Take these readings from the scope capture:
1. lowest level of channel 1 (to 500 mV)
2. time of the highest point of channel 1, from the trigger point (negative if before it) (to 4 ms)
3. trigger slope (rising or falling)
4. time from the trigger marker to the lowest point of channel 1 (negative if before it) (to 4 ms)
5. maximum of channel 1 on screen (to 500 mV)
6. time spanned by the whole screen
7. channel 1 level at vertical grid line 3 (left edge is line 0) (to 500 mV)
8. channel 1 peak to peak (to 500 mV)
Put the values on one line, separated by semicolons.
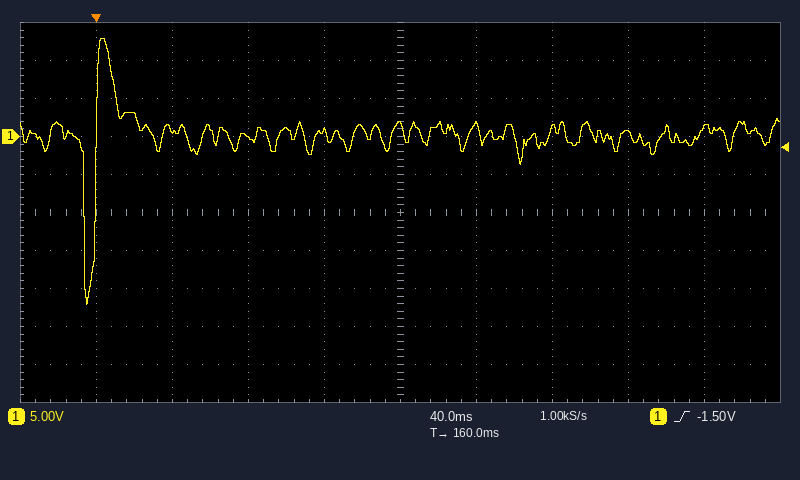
-22.0 V; +4 ms; rising; -4 ms; 13.0 V; 400 ms; 0.0 V; 35.0 V
